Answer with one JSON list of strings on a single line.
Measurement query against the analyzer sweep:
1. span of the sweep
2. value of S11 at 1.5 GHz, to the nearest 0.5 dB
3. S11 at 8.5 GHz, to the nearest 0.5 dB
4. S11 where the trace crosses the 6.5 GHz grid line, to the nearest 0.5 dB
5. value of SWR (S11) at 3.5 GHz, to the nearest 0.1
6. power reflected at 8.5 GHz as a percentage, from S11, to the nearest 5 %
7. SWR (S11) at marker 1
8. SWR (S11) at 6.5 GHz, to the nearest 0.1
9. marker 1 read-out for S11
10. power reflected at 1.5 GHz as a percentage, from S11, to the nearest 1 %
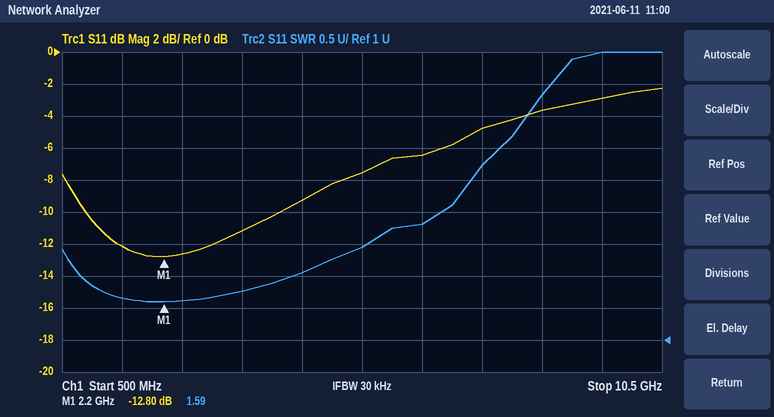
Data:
["10 GHz", "-12.0 dB", "-3.5 dB", "-6.5 dB", "1.8", "45 %", "1.59", "2.8", "-12.80 dB", "6 %"]
